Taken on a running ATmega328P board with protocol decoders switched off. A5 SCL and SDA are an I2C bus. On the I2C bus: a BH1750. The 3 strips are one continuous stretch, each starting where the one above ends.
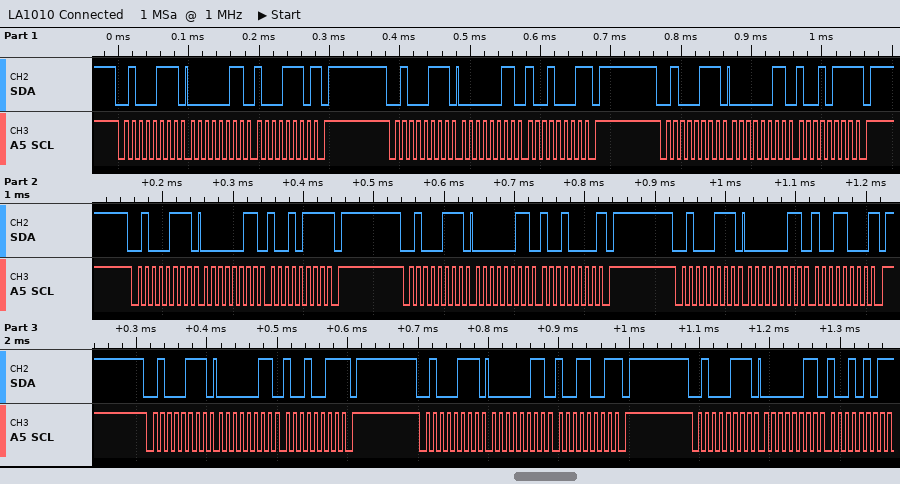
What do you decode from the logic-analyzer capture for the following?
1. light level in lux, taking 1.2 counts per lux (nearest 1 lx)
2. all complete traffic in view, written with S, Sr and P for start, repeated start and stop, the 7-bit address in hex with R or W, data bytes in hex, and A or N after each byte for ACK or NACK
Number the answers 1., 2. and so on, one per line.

1. 758 lx
2. S 23R A 03 A 8E N P S 23R A 03 A 91 N P S 23R A 03 A 97 N P S 23R A 03 A 97 N P S 23R A 03 A 90 N P S 23R A 03 A 98 N P S 23R A 03 A 93 N P S 23R A 03 A 99 N P S 23R A 03 A 95 N
